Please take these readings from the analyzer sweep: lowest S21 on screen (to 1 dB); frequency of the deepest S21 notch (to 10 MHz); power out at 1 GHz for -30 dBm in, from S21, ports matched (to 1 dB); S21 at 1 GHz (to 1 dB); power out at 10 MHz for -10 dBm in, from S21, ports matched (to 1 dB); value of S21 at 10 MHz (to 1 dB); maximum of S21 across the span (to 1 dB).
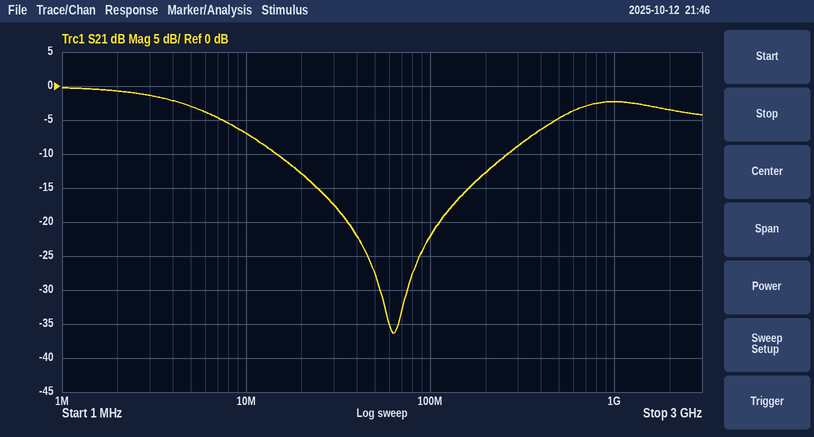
-36 dB
60 MHz
-32 dBm
-2 dB
-17 dBm
-7 dB
0 dB
